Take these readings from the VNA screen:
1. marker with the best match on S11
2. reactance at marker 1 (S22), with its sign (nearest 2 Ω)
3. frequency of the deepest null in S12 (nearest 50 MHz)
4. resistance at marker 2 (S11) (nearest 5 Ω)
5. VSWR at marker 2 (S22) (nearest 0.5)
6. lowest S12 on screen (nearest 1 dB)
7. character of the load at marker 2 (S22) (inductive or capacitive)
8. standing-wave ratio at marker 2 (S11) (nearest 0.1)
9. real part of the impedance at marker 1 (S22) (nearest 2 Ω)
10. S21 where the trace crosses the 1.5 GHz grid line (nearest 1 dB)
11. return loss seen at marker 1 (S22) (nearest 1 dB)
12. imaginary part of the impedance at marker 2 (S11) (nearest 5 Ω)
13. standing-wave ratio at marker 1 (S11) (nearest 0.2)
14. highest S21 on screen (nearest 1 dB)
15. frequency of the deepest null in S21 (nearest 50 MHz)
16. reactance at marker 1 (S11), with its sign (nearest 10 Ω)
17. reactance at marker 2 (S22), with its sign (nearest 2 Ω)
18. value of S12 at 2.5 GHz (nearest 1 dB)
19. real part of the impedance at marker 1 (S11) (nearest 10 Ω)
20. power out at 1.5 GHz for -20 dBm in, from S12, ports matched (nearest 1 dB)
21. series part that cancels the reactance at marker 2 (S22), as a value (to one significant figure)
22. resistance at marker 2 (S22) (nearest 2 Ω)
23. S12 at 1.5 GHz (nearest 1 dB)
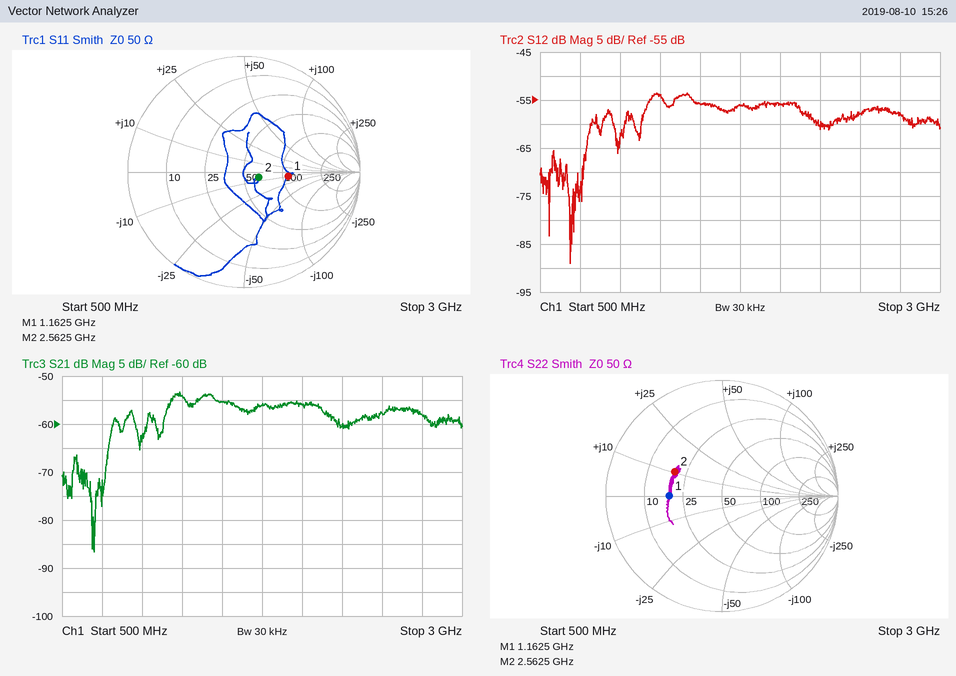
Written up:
marker 2
0 Ω
700 MHz
65 Ω
2.5
-89 dB
inductive
1.3
18 Ω
-55 dB
7 dB
-5 Ω
2.2
-53 dB
700 MHz
-10 Ω
+10 Ω
-58 dB
110 Ω
-76 dBm
6 pF
20 Ω
-56 dB
